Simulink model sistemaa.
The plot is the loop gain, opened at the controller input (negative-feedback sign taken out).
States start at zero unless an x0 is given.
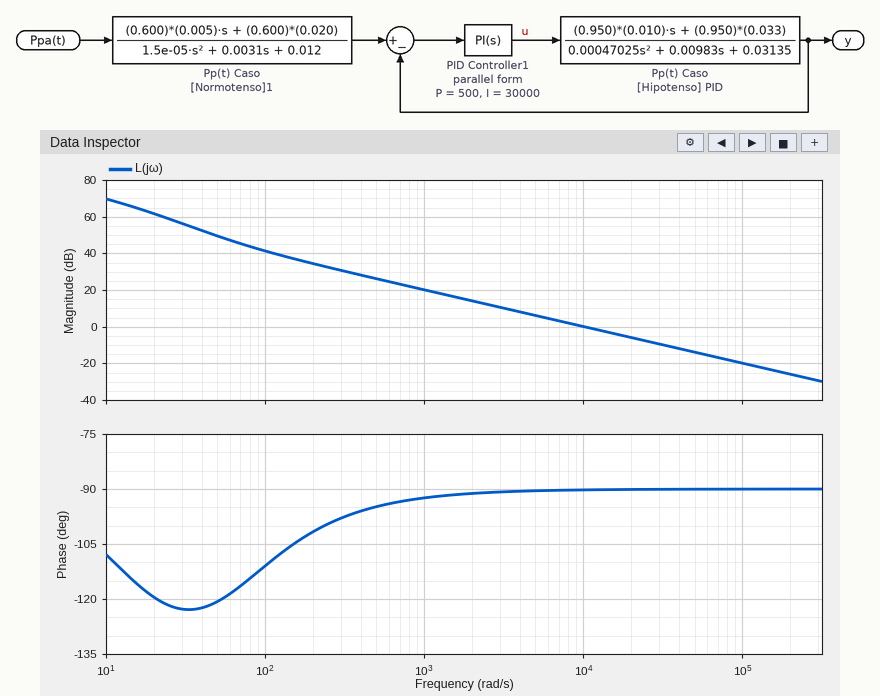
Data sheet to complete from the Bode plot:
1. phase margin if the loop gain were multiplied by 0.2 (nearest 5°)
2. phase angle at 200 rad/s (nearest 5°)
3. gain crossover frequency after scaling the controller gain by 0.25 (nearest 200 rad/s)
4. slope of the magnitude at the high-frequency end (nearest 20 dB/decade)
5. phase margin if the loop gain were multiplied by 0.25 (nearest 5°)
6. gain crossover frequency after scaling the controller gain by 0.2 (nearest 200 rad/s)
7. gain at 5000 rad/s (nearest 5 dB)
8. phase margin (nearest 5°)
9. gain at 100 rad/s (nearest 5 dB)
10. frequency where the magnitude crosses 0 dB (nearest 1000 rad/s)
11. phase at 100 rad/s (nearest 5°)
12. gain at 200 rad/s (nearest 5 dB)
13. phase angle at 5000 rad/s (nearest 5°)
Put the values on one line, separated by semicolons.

90°; -100°; 2600 rad/s; -20 dB/decade; 90°; 2000 rad/s; 5 dB; 90°; 40 dB; 10000 rad/s; -110°; 35 dB; -90°
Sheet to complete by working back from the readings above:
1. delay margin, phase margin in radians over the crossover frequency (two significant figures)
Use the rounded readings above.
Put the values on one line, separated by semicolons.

0.00016 s
